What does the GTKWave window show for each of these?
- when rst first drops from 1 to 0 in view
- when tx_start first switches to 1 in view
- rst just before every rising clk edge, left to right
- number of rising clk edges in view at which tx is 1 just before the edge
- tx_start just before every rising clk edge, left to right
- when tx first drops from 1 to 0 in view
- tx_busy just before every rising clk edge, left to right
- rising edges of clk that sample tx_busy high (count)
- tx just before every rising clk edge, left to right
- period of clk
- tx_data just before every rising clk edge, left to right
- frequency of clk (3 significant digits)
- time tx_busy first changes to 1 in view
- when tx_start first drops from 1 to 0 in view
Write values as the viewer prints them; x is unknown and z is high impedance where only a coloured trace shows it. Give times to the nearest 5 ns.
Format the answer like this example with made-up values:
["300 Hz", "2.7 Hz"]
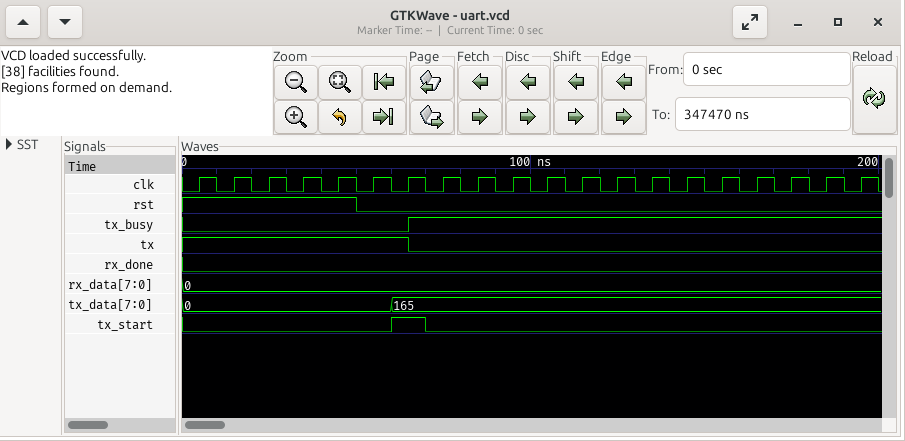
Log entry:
["50 ns", "60 ns", "1 1 1 1 1 0 0 0 0 0 0 0 0 0 0 0 0 0 0 0", "7", "0 0 0 0 0 0 1 0 0 0 0 0 0 0 0 0 0 0 0 0", "65 ns", "0 0 0 0 0 0 0 1 1 1 1 1 1 1 1 1 1 1 1 1", "13", "1 1 1 1 1 1 1 0 0 0 0 0 0 0 0 0 0 0 0 0", "10 ns", "0, 0, 0, 0, 0, 0, 165, 165, 165, 165, 165, 165, 165, 165, 165, 165, 165, 165, 165, 165", "100 MHz", "65 ns", "70 ns"]
